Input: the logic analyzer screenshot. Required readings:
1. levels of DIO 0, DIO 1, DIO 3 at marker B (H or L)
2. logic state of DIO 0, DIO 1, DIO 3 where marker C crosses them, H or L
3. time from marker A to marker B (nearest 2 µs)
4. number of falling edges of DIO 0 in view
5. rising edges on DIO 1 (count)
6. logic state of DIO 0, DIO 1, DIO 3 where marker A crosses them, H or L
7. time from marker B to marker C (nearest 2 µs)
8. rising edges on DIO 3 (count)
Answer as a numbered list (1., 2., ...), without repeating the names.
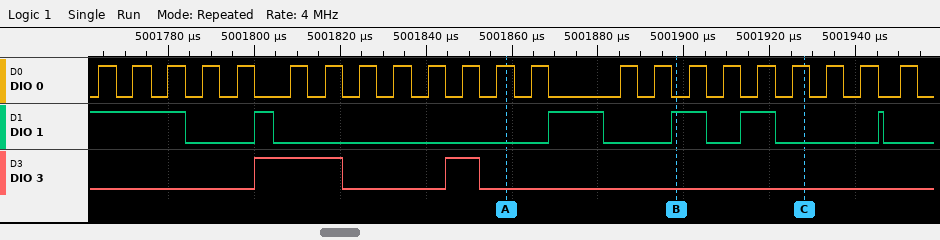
1. DIO 0=L, DIO 1=H, DIO 3=L
2. DIO 0=H, DIO 1=L, DIO 3=L
3. 40 µs
4. 22
5. 5
6. DIO 0=H, DIO 1=L, DIO 3=L
7. 30 µs
8. 2
